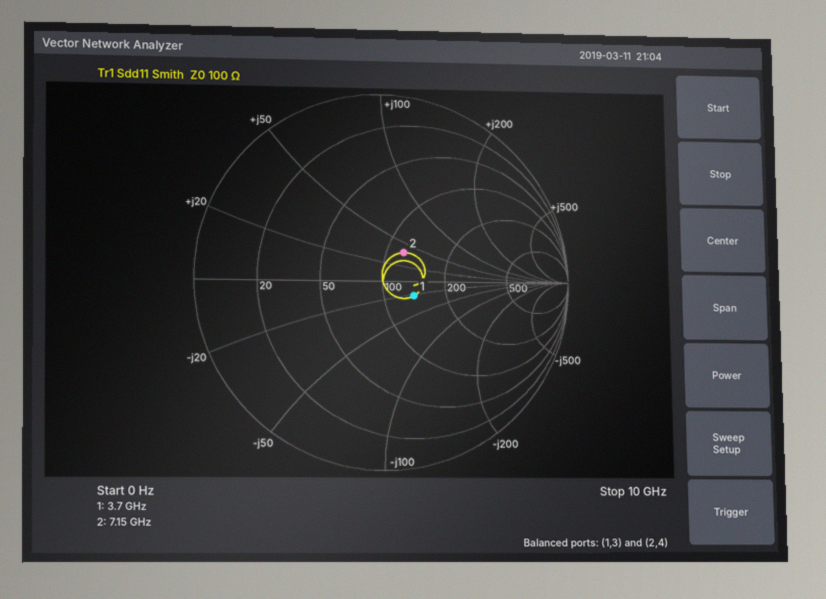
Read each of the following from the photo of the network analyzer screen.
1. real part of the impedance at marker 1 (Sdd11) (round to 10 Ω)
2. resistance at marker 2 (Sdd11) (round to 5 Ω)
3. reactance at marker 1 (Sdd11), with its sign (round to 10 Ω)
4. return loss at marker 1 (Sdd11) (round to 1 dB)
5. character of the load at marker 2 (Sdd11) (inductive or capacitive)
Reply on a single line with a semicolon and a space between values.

140 Ω; 120 Ω; -20 Ω; 15 dB; inductive
